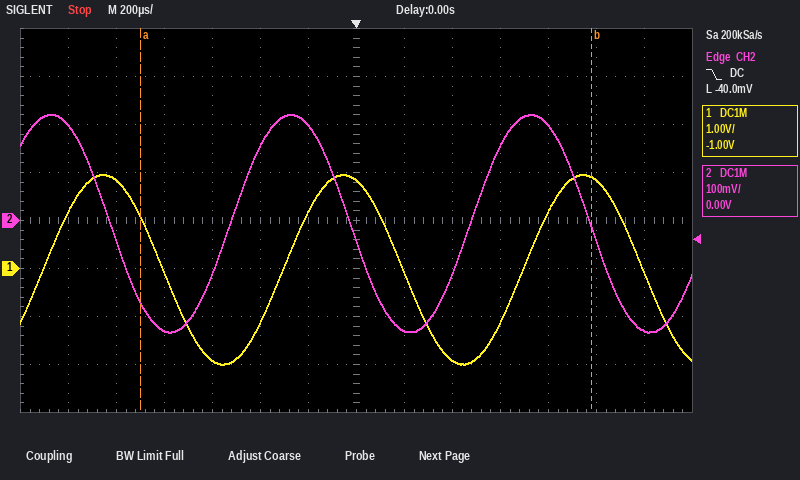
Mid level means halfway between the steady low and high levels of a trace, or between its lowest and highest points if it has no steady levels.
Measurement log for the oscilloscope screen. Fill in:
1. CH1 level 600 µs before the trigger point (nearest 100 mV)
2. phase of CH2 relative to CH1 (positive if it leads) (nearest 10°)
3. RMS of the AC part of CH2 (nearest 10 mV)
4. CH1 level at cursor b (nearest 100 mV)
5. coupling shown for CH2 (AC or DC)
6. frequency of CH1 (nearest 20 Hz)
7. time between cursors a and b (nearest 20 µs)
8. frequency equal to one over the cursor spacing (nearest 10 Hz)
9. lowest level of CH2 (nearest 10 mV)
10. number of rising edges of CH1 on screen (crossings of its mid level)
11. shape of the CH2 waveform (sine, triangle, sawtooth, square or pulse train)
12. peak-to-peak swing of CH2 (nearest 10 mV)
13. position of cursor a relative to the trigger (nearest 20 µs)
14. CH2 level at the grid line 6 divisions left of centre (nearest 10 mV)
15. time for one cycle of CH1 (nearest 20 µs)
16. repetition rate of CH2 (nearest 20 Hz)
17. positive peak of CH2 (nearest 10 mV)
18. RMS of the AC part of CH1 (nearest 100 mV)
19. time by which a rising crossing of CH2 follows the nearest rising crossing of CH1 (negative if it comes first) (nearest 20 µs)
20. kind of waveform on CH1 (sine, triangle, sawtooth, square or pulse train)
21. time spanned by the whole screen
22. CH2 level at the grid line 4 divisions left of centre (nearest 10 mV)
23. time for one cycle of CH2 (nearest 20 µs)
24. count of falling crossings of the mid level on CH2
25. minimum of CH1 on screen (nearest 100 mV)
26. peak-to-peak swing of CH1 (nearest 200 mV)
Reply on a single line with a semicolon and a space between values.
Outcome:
-1.9 V; +80°; 160 mV; 1.9 V; DC; 1.00 kHz; 1.88 ms; 530 Hz; -230 mV; 3; sine; 450 mV; -900 µs; 200 mV; 1.00 ms; 1.00 kHz; 220 mV; 1.4 V; -220 µs; sine; 2.8 ms; -230 mV; 1.00 ms; 3; -2.0 V; 4.0 V
